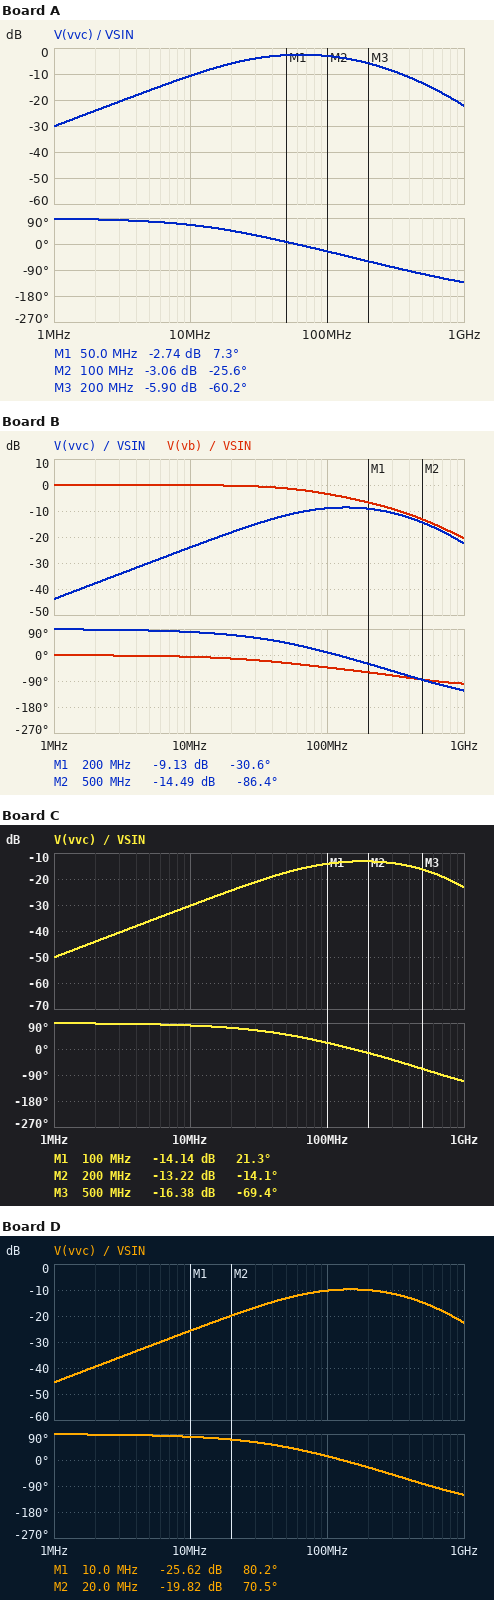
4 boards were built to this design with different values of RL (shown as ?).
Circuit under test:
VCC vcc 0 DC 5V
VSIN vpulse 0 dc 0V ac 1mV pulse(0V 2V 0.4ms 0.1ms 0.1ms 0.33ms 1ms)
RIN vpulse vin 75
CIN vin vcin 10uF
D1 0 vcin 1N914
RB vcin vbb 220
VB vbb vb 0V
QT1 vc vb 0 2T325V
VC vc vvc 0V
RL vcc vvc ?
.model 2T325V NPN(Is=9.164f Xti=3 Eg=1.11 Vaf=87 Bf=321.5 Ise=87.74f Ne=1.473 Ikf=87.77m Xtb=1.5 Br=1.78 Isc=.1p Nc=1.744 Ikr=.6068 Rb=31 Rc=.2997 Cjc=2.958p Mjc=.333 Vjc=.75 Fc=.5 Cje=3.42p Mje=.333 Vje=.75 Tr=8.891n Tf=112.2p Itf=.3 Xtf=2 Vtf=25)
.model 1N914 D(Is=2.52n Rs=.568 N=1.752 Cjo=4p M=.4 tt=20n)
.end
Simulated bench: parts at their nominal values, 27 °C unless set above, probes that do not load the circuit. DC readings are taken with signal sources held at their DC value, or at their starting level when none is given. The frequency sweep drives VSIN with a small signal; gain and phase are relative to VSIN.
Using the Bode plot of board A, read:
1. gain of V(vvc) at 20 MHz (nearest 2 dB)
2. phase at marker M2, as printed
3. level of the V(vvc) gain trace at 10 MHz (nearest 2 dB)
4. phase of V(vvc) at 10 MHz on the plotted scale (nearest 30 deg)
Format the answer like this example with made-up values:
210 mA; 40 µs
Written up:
-6 dB; -25.6 deg; -10 dB; 60 deg
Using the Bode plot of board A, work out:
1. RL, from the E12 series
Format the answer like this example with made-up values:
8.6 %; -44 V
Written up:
3.3 kΩ
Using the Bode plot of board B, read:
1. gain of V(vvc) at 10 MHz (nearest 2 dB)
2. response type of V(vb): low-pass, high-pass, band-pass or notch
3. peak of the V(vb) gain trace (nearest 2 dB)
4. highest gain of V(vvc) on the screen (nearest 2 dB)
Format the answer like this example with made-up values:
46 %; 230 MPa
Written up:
-24 dB; low-pass; 0 dB; -8 dB
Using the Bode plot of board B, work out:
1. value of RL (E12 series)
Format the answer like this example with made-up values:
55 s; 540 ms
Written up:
680 Ω
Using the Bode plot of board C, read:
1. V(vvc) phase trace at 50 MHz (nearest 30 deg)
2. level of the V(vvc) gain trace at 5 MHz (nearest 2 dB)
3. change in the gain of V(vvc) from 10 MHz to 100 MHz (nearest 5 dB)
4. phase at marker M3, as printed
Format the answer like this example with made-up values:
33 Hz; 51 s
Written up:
60 deg; -36 dB; 15 dB; -69.4 deg
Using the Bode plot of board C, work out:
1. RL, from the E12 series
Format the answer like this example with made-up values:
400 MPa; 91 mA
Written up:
330 Ω
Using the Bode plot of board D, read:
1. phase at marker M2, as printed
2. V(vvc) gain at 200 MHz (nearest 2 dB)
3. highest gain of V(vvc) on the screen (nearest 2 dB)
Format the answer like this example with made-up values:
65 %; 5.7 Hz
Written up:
70.5 deg; -10 dB; -10 dB
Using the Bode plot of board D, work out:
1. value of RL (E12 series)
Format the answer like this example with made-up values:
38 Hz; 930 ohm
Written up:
560 Ω
